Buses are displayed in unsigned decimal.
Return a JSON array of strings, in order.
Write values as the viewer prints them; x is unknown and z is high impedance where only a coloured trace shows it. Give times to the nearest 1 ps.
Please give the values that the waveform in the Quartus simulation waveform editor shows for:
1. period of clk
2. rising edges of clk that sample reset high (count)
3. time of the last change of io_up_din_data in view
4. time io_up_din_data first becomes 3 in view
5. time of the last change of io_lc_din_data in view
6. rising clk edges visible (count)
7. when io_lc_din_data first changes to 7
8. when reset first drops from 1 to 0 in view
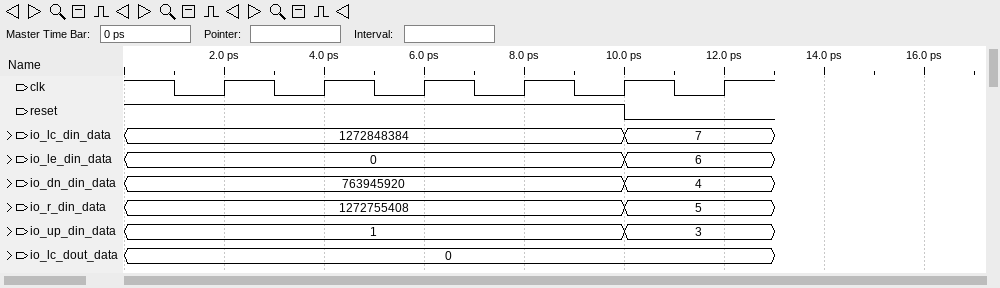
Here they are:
["2 ps", "5", "10 ps", "10 ps", "10 ps", "6", "10 ps", "10 ps"]
